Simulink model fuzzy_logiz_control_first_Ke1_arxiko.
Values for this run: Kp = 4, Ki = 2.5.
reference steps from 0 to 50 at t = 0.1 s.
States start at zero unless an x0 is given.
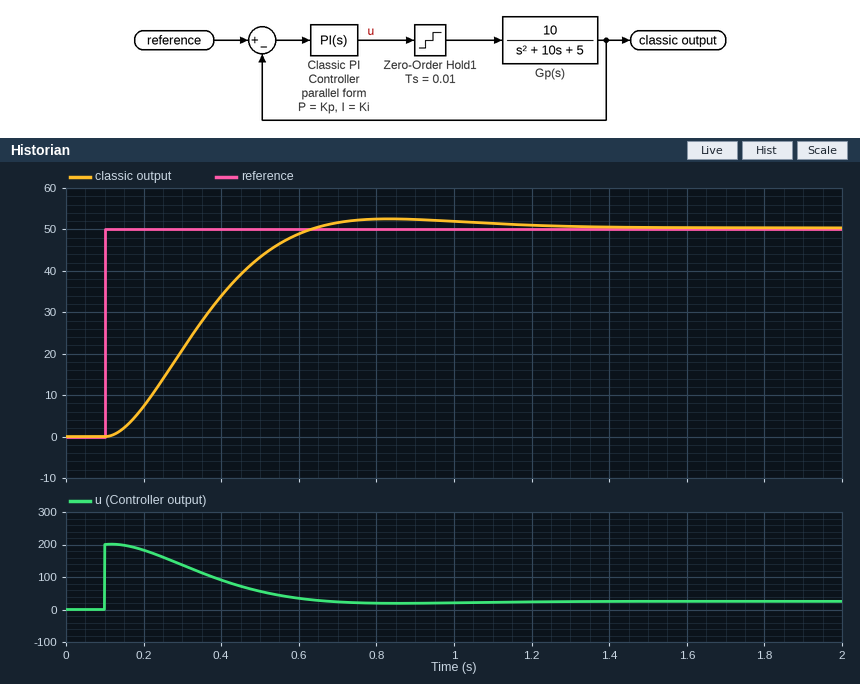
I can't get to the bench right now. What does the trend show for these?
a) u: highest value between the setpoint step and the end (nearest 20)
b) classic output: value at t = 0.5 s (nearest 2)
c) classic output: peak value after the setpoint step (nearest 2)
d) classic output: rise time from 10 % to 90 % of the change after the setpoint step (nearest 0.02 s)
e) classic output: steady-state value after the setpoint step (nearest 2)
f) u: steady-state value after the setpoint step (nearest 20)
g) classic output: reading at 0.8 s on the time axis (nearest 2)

200
44
52
0.34 s
50
20
52
